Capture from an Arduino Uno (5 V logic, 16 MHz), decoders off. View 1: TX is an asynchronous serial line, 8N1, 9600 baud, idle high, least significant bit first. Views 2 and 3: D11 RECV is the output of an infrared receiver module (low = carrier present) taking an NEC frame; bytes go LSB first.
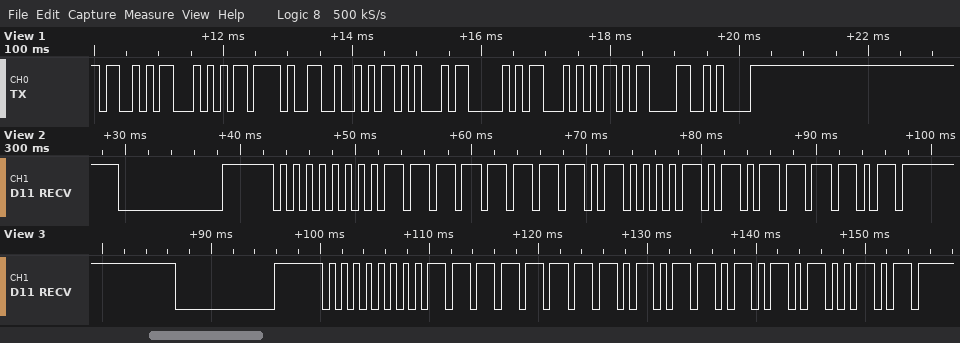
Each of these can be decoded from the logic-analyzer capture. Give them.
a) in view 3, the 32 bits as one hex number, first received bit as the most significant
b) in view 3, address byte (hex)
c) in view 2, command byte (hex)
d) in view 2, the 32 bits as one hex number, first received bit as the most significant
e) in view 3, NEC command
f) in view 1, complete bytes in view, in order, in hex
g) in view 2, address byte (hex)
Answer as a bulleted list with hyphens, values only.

- 0x00FF5AA5
- 0x00
- 0x42
- 0x00FF42BD
- 0x5A
- 0x53 0x54 0x2F 0x52 0x45 0x50 0x54 0x0D 0x0A
- 0x00
